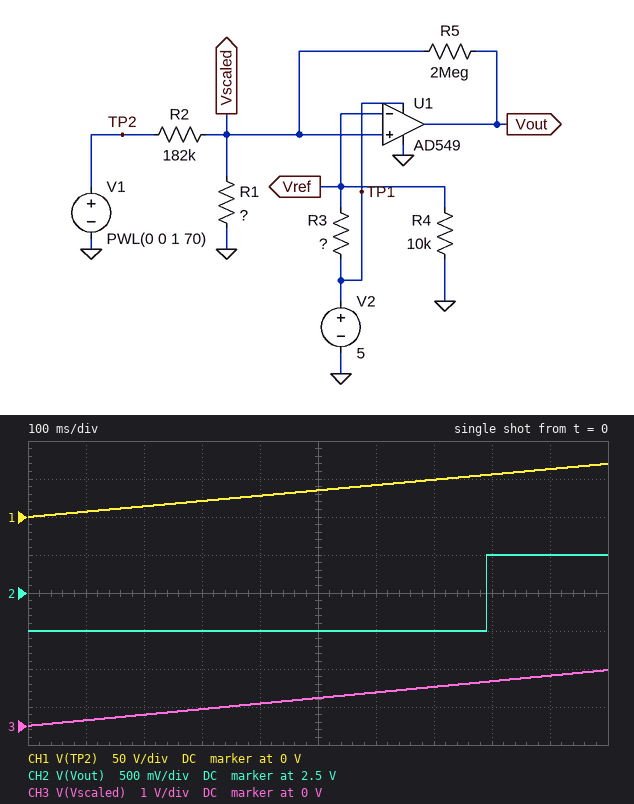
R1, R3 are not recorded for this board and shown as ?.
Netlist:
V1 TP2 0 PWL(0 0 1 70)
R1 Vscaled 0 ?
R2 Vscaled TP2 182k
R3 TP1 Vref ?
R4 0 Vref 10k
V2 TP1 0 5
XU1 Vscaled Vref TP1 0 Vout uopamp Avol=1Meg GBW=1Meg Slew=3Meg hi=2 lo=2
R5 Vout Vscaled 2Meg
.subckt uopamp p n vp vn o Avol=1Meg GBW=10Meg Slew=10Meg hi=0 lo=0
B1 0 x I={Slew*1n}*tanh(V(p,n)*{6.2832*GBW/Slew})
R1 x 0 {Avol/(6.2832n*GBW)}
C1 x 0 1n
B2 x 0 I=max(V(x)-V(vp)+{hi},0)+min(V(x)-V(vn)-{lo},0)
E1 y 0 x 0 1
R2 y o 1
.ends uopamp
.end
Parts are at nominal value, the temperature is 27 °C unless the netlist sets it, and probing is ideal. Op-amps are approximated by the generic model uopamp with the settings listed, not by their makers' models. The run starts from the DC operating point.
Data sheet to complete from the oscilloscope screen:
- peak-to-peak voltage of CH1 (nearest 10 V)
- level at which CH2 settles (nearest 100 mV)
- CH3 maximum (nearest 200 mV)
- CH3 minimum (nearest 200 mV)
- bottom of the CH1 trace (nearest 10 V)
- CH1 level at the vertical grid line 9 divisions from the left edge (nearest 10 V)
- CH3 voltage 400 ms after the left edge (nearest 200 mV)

70 V
3.0 V
1.4 V
0 V
0 V
60 V
600 mV
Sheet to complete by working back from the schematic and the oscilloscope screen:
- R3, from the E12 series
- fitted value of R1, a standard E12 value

33 kΩ
3.9 kΩ
